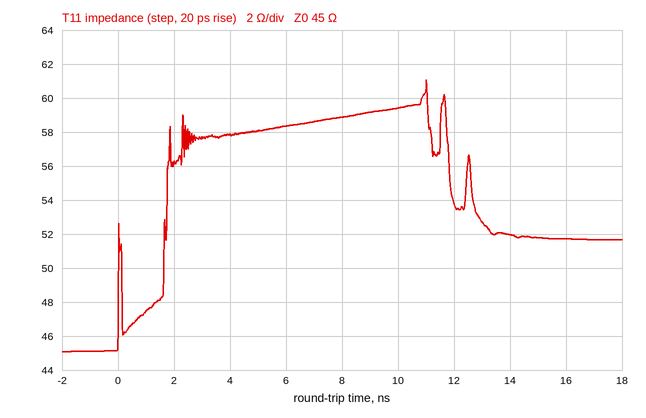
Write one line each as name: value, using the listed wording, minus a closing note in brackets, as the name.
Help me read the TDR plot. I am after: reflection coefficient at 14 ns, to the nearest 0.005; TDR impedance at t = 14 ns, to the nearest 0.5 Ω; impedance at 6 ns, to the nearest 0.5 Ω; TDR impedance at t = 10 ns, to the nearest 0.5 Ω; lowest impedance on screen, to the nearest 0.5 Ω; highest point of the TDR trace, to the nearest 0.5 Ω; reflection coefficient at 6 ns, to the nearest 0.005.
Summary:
reflection coefficient at 14 ns, to the nearest 0.005: +0.070
TDR impedance at t = 14 ns, to the nearest 0.5 Ω: 52.0 Ω
impedance at 6 ns, to the nearest 0.5 Ω: 58.5 Ω
TDR impedance at t = 10 ns, to the nearest 0.5 Ω: 59.5 Ω
lowest impedance on screen, to the nearest 0.5 Ω: 45.0 Ω
highest point of the TDR trace, to the nearest 0.5 Ω: 61.0 Ω
reflection coefficient at 6 ns, to the nearest 0.005: +0.130
